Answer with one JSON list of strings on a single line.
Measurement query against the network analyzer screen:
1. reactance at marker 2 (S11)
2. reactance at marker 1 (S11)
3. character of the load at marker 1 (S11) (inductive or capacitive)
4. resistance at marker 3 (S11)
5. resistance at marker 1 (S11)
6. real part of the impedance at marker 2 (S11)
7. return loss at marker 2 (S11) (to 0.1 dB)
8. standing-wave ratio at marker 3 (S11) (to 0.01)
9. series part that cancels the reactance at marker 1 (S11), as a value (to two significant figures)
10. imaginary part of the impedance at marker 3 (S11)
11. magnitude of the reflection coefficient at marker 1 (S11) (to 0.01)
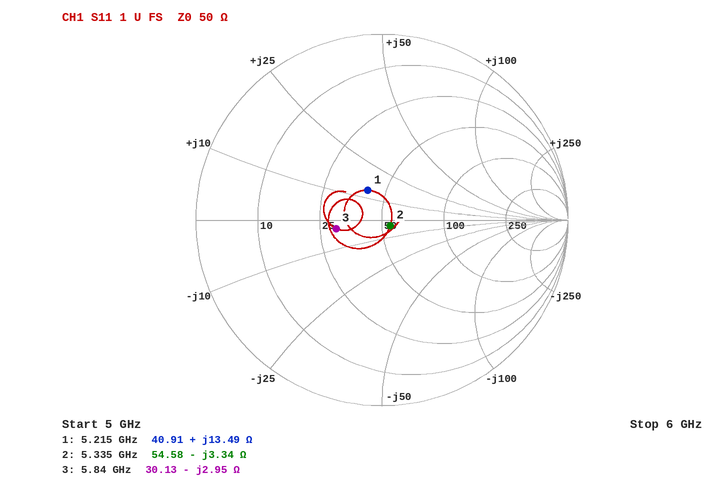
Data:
["-3.34 Ω", "+13.49 Ω", "inductive", "30.13 Ω", "40.91 Ω", "54.58 Ω", "25.3 dB", "1.67", "2.3 pF", "-2.95 Ω", "0.18"]
